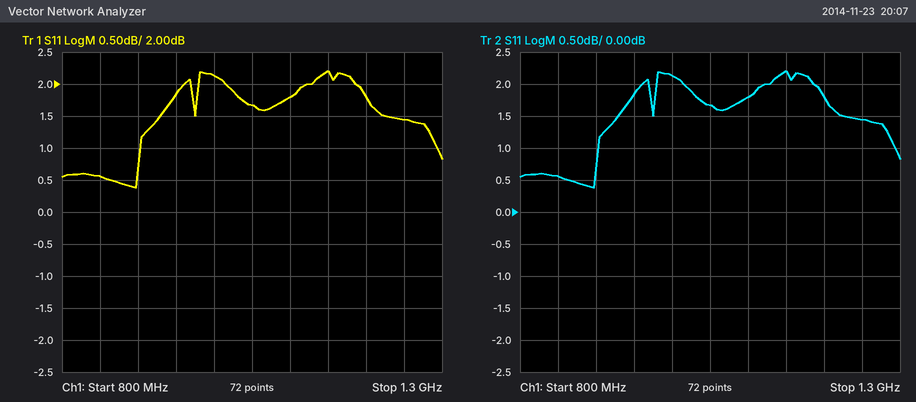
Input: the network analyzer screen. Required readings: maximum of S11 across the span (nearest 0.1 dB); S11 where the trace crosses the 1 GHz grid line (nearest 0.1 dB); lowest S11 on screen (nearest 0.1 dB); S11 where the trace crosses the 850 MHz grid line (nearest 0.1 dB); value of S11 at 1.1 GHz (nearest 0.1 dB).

2.2 dB
2.1 dB
0.4 dB
0.6 dB
1.8 dB
